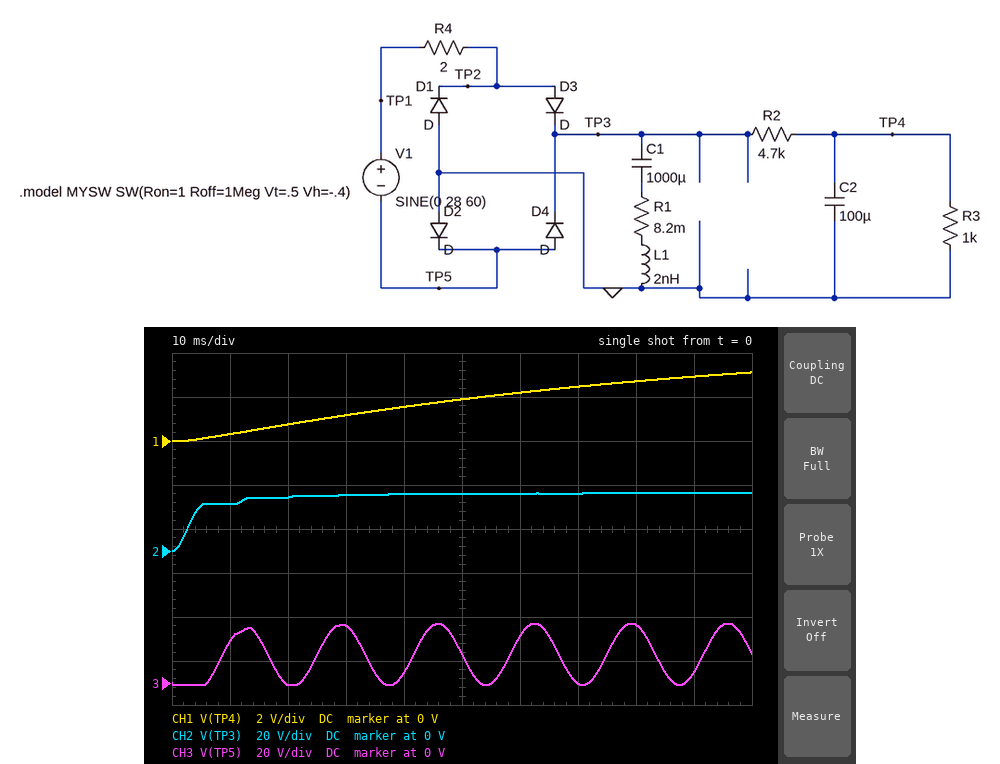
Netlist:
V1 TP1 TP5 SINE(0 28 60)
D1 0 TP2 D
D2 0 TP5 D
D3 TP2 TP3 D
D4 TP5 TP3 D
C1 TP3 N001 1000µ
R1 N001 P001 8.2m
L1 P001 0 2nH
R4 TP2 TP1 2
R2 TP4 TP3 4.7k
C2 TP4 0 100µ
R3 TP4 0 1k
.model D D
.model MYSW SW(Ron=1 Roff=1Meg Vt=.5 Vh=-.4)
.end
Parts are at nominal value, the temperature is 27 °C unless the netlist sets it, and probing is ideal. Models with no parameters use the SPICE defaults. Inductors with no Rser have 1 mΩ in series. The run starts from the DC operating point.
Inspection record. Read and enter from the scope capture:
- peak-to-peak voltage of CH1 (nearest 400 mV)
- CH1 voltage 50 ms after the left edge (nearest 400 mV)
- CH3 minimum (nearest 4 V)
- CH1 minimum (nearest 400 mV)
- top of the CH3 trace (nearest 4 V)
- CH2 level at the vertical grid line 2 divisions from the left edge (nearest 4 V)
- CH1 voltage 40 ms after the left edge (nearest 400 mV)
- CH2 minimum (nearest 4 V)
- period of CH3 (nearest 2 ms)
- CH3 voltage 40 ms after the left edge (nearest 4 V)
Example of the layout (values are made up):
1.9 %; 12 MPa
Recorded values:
3.2 V; 2.0 V; 0 V; 0 V; 28 V; 24 V; 1.6 V; 0 V; 16 ms; 4 V
